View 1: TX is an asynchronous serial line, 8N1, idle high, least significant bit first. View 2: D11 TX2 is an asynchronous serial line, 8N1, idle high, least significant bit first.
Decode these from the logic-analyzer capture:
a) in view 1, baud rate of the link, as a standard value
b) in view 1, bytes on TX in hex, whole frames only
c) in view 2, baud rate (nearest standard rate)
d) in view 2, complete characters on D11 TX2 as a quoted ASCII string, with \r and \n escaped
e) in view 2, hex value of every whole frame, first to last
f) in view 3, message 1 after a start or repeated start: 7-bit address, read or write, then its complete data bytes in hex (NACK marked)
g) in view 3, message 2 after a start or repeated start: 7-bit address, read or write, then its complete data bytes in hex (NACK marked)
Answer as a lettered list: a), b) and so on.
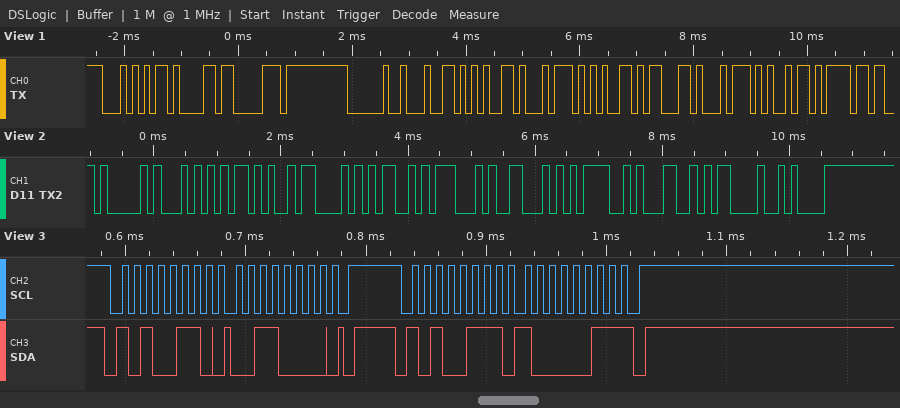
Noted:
a) 9600 baud
b) 54 61 70 20 64 65 74 65 63 74 69 6F
c) 9600 baud
d) "AT+CMGF=1\r\n"
e) 41 54 2B 43 4D 47 46 3D 31 0D 0A
f) 0x53 write: 30
g) 0x53 read: 83 NACK
